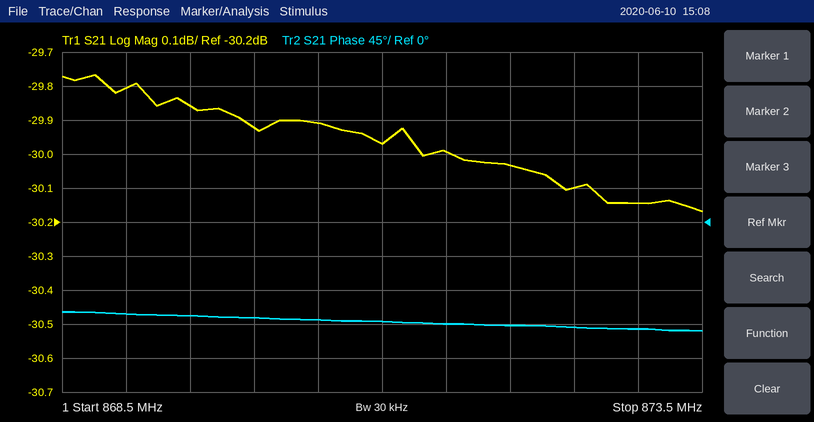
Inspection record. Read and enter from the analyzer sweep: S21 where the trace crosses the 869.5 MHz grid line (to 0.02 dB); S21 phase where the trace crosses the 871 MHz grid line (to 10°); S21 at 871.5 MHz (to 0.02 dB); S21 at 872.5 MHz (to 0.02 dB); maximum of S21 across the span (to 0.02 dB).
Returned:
-29.86 dB
-130°
-30.00 dB
-30.10 dB
-29.76 dB
